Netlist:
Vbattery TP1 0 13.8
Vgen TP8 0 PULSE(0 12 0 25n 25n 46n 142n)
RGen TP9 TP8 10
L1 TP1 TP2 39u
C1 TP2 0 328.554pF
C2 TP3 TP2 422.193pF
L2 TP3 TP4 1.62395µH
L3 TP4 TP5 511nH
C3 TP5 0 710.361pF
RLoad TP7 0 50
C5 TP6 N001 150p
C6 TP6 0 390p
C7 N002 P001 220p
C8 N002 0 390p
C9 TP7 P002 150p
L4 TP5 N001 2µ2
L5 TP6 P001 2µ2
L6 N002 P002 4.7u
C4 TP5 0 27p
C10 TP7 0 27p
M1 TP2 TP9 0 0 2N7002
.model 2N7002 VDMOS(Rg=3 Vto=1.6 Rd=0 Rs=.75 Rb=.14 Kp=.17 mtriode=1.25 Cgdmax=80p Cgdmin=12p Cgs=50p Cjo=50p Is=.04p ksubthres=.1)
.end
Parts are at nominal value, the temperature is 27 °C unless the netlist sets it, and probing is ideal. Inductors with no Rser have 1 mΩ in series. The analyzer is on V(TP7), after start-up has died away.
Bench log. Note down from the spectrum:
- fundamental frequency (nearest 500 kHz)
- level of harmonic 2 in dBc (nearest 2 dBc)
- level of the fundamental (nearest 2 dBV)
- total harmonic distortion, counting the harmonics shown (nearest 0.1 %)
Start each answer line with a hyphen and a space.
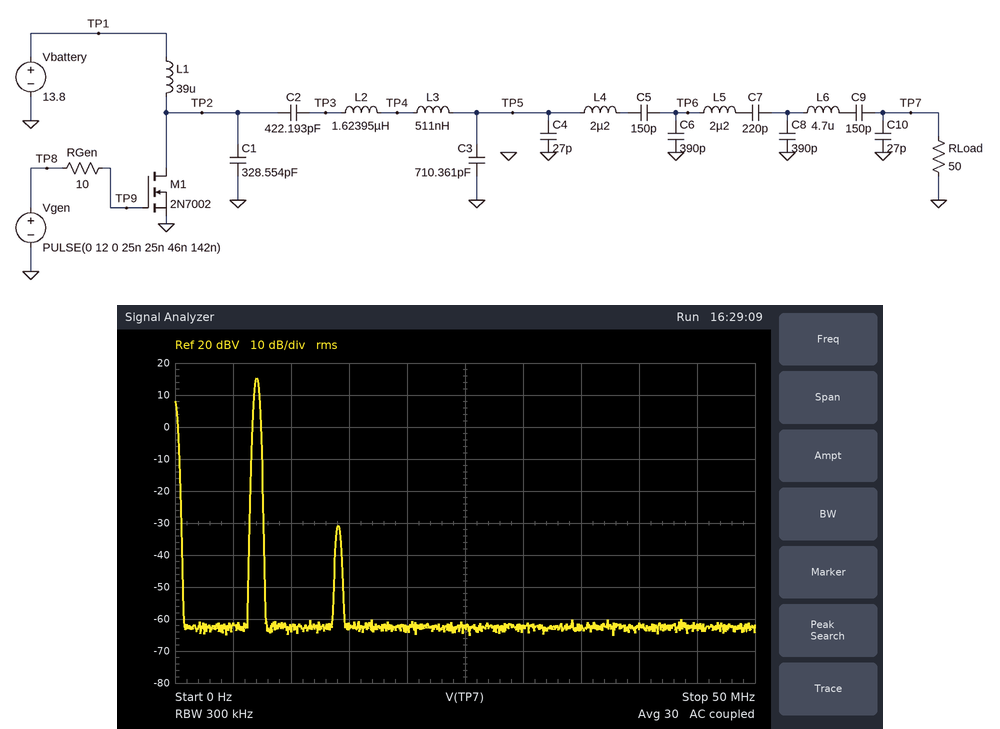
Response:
- 7.0 MHz
- -46 dBc
- 16 dBV
- 0.5 %
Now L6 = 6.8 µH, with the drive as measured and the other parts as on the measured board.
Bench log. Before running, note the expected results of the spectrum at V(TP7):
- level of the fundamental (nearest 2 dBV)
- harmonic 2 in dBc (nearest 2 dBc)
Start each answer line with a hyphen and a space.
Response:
- 8 dBV
- -44 dBc
